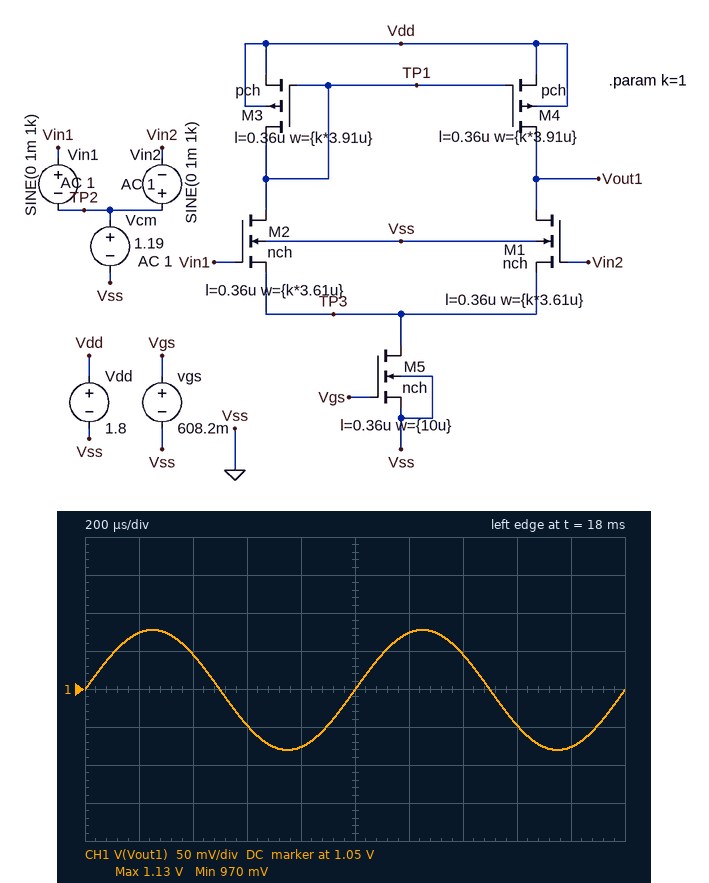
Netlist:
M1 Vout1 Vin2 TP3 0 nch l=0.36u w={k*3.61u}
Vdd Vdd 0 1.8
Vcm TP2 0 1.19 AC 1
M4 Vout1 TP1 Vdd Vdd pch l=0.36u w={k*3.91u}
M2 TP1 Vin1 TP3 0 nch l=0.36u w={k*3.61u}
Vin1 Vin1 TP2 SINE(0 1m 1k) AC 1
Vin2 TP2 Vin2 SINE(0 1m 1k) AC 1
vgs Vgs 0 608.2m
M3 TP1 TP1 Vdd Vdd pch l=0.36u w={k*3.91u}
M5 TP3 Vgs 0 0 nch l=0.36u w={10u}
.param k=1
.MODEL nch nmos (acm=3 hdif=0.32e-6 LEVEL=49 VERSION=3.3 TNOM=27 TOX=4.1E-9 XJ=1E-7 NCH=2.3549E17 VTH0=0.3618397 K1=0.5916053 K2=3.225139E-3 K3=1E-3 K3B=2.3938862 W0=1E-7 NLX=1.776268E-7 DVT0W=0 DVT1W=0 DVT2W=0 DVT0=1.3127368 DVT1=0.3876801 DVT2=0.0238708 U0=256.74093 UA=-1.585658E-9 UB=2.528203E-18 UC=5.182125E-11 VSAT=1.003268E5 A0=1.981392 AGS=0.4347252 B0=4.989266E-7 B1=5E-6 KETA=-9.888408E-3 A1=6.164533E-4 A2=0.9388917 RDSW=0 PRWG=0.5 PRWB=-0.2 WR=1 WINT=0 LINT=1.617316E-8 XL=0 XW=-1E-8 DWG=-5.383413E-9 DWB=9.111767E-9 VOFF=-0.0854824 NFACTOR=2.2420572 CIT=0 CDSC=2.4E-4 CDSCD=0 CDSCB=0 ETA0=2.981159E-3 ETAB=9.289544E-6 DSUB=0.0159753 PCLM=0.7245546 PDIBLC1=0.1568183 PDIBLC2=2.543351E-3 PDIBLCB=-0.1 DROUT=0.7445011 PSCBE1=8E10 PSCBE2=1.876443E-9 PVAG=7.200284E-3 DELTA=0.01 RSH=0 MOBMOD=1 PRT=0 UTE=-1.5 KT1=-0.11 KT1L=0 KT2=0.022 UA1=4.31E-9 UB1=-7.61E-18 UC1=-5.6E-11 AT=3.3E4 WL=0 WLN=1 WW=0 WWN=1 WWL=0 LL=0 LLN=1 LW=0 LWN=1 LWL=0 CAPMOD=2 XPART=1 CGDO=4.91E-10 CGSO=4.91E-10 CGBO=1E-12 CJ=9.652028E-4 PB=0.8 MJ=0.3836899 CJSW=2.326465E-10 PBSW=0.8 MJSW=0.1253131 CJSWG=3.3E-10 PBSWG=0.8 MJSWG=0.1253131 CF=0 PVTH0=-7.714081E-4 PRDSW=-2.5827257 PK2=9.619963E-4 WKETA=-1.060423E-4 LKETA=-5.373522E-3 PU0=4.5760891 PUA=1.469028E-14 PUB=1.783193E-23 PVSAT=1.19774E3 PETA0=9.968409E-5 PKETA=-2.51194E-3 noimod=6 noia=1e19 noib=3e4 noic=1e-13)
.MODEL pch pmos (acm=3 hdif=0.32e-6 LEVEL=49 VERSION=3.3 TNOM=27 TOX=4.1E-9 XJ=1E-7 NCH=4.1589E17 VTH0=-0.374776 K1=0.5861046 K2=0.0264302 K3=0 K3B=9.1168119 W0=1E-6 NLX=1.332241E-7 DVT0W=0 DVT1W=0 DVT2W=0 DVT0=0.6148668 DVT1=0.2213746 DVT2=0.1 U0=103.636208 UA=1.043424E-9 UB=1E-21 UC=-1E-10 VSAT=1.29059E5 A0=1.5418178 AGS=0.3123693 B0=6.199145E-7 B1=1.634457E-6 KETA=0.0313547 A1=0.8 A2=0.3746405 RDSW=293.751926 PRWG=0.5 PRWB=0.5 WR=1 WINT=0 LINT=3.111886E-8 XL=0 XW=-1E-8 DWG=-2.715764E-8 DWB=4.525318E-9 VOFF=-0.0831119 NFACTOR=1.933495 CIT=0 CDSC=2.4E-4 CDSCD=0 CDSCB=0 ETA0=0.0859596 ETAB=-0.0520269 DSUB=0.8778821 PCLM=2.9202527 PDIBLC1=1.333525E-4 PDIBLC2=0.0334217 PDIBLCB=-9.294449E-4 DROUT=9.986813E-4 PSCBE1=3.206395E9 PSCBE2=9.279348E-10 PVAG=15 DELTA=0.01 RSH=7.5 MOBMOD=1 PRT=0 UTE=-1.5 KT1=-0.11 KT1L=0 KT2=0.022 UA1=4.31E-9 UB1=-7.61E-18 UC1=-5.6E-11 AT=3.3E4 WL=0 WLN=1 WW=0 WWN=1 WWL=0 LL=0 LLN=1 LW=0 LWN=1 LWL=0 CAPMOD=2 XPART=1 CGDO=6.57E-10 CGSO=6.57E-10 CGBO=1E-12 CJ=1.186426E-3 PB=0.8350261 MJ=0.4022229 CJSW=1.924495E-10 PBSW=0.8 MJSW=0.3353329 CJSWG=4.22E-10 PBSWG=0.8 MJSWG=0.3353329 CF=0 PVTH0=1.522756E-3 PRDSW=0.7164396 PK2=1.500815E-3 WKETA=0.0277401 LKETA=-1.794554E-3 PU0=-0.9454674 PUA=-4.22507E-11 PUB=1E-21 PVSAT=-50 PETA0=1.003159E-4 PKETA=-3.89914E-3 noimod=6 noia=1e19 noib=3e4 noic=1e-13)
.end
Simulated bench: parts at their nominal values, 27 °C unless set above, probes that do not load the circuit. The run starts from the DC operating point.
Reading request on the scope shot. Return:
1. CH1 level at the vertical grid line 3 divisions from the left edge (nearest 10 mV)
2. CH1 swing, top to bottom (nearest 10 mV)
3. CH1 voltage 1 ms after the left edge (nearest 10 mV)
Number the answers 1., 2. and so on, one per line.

1. 1.00 V
2. 160 mV
3. 1.05 V
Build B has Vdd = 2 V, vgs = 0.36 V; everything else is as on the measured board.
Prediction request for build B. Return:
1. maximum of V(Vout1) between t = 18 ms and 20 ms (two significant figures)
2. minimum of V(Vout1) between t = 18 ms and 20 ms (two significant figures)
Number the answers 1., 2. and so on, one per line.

1. 1.7 V
2. 1.5 V
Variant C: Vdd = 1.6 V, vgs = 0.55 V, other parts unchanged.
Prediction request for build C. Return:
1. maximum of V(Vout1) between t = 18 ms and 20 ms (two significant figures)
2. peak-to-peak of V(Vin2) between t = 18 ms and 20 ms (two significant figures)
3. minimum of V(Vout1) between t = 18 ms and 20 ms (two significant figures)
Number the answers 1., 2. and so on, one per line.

1. 1.0 V
2. 2.0 mV
3. 880 mV
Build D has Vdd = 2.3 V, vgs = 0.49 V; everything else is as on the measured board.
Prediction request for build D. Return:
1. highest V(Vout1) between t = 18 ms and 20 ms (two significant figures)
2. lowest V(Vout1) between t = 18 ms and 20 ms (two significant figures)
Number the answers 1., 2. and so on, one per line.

1. 1.8 V
2. 1.7 V
